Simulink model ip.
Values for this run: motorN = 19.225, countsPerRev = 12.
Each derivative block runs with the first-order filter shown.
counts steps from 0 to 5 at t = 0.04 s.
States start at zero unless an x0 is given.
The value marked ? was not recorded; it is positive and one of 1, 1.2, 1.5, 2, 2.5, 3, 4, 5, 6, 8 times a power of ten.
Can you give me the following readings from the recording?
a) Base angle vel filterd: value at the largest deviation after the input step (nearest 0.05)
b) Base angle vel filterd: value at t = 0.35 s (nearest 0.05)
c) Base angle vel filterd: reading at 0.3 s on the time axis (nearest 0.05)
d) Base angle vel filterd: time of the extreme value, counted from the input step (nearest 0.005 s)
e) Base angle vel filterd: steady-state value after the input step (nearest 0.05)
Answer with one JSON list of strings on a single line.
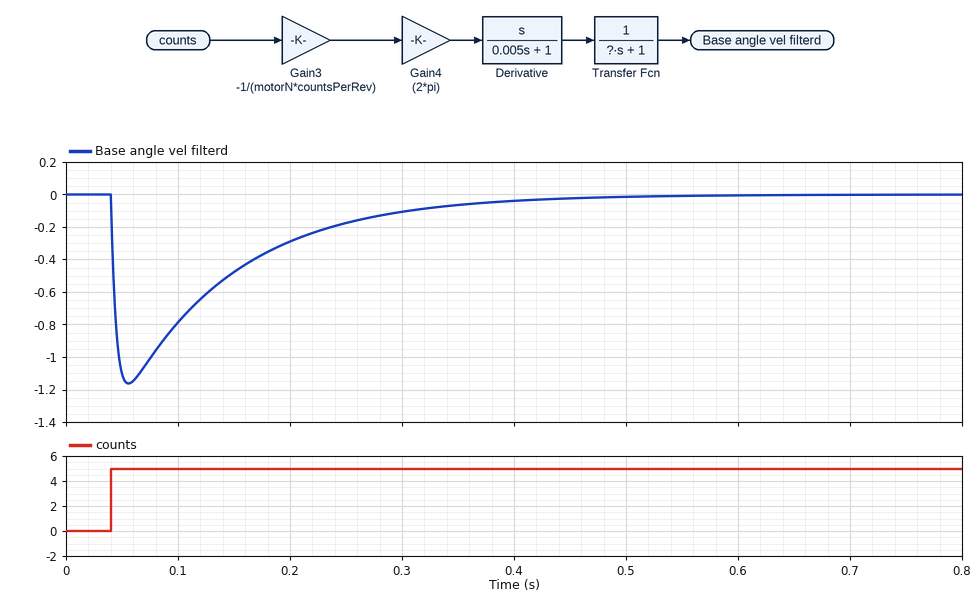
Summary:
["-1.15", "-0.05", "-0.10", "0.015 s", "0.00"]
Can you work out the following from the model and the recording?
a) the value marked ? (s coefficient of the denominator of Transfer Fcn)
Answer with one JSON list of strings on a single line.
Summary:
["0.1"]
